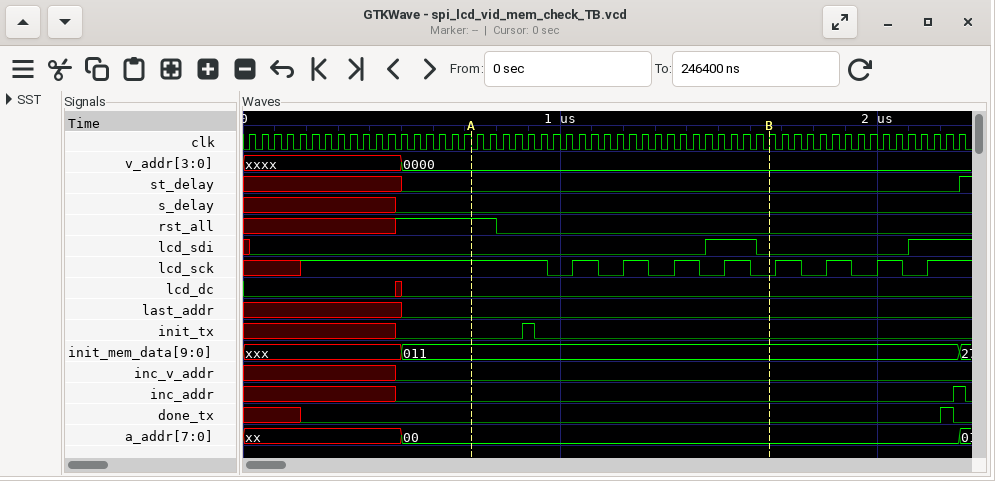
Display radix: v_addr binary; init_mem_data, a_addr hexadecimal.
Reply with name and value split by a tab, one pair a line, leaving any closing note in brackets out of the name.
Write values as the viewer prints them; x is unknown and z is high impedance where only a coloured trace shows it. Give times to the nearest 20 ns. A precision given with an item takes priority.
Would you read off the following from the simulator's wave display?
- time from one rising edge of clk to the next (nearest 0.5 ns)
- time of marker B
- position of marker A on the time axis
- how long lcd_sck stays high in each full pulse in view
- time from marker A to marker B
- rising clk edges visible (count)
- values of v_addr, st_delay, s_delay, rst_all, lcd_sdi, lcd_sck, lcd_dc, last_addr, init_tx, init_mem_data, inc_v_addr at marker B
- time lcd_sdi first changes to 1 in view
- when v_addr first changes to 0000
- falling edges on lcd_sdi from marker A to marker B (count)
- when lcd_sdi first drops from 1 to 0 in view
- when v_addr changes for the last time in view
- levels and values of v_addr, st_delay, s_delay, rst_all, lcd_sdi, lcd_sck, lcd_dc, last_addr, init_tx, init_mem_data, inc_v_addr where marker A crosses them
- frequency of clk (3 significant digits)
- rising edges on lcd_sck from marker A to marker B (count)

time from one rising edge of clk to the next	40 ns
time of marker B	1660 ns
position of marker A on the time axis	720 ns
how long lcd_sck stays high in each full pulse in view	80 ns, 80 ns, 80 ns, 80 ns, 80 ns, 80 ns, 80 ns
time from marker A to marker B	940 ns
rising clk edges visible	57
values of v_addr, st_delay, s_delay, rst_all, lcd_sdi, lcd_sck, lcd_dc, last_addr, init_tx, init_mem_data, inc_v_addr at marker B	v_addr=0000, st_delay=0, s_delay=0, rst_all=0, lcd_sdi=0, lcd_sck=0, lcd_dc=0, last_addr=0, init_tx=0, init_mem_data=011, inc_v_addr=0
time lcd_sdi first changes to 1 in view	1460 ns
when v_addr first changes to 0000	500 ns
falling edges on lcd_sdi from marker A to marker B	1
when lcd_sdi first drops from 1 to 0 in view	1620 ns
when v_addr changes for the last time in view	500 ns
levels and values of v_addr, st_delay, s_delay, rst_all, lcd_sdi, lcd_sck, lcd_dc, last_addr, init_tx, init_mem_data, inc_v_addr where marker A crosses them	v_addr=0000, st_delay=0, s_delay=0, rst_all=1, lcd_sdi=0, lcd_sck=1, lcd_dc=0, last_addr=0, init_tx=0, init_mem_data=011, inc_v_addr=0
frequency of clk	25.0 MHz
rising edges on lcd_sck from marker A to marker B	4
